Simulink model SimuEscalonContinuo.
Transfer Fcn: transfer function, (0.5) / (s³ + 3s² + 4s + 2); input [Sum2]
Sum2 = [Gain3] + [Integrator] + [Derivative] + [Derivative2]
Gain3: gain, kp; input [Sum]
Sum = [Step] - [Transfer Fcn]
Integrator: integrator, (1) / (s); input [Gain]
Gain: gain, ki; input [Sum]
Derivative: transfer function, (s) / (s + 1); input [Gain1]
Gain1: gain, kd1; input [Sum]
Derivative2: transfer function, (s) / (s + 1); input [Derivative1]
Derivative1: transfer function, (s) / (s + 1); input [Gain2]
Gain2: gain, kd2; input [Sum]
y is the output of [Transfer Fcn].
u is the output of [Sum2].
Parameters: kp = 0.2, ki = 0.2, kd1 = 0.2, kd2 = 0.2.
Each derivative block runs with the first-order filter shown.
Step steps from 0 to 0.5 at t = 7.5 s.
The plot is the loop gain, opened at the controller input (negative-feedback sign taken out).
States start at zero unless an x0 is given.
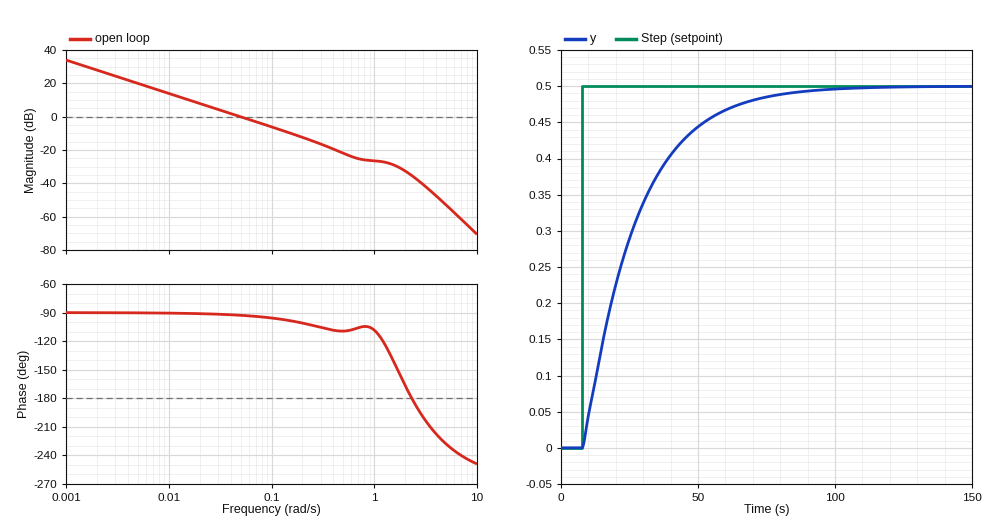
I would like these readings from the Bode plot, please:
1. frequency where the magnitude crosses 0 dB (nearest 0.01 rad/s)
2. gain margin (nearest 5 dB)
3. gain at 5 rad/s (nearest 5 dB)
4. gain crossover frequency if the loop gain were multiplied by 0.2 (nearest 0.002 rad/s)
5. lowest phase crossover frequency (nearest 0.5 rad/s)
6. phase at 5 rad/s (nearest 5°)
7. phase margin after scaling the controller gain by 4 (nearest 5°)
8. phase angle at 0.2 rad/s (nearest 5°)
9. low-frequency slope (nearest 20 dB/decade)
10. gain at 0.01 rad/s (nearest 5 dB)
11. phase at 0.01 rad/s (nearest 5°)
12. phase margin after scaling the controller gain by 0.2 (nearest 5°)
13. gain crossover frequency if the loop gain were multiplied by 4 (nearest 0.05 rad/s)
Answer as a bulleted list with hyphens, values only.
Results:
- 0.05 rad/s
- 35 dB
- -55 dB
- 0.010 rad/s
- 2.5 rad/s
- -230°
- 80°
- -100°
- -20 dB/decade
- 15 dB
- -90°
- 90°
- 0.20 rad/s
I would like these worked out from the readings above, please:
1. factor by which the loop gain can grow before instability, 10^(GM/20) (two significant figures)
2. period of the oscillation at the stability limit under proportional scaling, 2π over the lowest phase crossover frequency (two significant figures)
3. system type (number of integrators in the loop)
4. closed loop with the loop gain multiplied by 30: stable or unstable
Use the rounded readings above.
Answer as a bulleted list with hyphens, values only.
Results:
- 56
- 2.5 s
- 1
- stable
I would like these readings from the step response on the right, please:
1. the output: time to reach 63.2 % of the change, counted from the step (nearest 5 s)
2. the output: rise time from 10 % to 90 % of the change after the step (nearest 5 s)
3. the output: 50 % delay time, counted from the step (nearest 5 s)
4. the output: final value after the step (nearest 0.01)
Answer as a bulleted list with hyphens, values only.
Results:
- 20 s
- 40 s
- 15 s
- 0.50
